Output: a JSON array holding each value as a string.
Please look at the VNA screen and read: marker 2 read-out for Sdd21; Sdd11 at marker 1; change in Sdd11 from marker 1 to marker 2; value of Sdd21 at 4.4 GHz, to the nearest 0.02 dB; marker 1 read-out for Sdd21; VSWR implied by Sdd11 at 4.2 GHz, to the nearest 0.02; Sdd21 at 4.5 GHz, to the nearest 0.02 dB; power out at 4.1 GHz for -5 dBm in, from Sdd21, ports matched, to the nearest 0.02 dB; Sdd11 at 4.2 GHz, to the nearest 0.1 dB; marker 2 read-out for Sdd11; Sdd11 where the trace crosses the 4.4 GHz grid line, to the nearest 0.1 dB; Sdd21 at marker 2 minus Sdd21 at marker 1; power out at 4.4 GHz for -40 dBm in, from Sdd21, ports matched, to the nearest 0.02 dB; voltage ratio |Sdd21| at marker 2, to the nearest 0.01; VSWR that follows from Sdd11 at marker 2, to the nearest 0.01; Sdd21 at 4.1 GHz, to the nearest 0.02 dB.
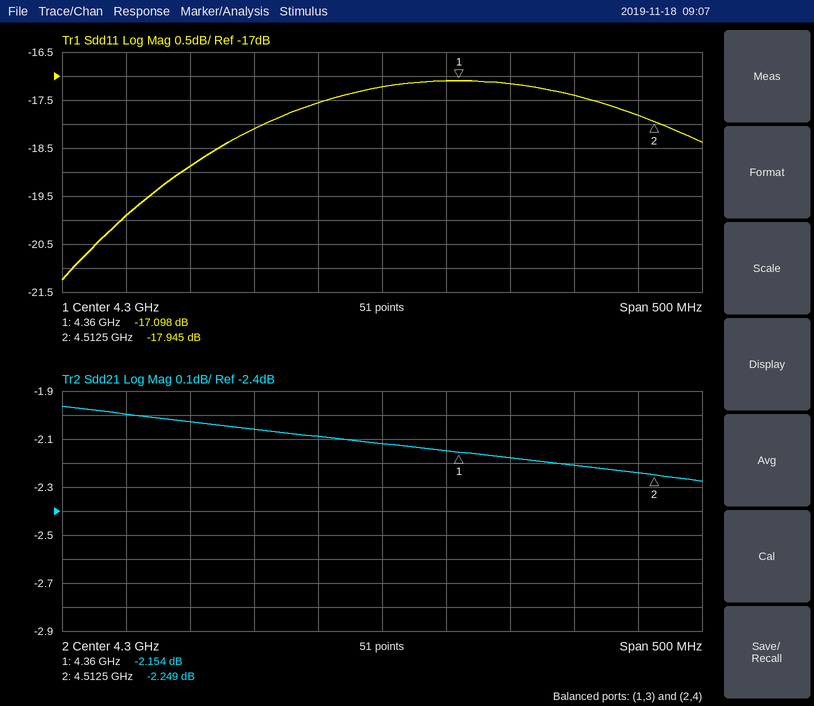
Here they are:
["-2.249 dB", "-17.098 dB", "-0.847 dB", "-2.18 dB", "-2.154 dB", "1.28", "-2.24 dB", "-7.00 dBm", "-18.1 dB", "-17.945 dB", "-17.2 dB", "-0.095 dB", "-42.18 dBm", "0.77", "1.29", "-2.00 dB"]
